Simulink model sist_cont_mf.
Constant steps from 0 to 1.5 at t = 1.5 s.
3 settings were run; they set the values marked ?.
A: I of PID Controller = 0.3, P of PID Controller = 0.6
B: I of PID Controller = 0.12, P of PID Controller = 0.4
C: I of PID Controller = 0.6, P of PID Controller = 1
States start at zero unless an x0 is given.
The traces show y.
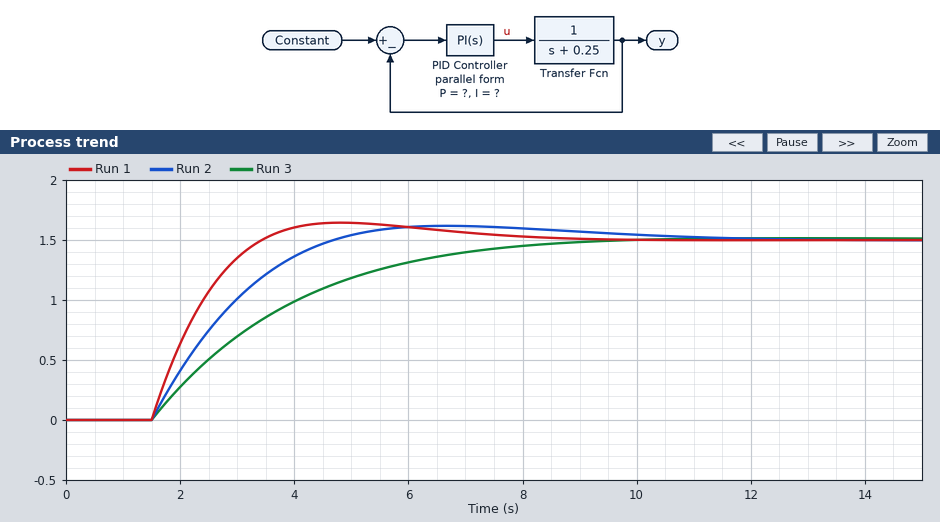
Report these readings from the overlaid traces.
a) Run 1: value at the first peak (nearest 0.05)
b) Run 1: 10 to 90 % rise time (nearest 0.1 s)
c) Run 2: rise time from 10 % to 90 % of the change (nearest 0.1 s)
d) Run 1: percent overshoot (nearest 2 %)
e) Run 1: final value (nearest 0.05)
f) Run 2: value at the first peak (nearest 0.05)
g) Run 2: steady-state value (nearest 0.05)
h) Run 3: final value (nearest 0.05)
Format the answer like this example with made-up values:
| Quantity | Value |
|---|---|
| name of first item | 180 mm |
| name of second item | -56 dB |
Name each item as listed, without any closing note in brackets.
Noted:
| Quantity | Value |
|---|---|
| Run 1: value at the first peak | 1.65 |
| Run 1: 10 to 90 % rise time | 1.4 s |
| Run 2: rise time from 10 % to 90 % of the change | 2.3 s |
| Run 1: percent overshoot | 10 % |
| Run 1: final value | 1.50 |
| Run 2: value at the first peak | 1.60 |
| Run 2: steady-state value | 1.50 |
| Run 3: final value | 1.50 |
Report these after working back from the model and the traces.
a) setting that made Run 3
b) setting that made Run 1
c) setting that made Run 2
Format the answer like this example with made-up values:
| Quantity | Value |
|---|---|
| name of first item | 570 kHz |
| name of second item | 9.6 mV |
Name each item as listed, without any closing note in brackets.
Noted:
| Quantity | Value |
|---|---|
| setting that made Run 3 | B |
| setting that made Run 1 | C |
| setting that made Run 2 | A |
